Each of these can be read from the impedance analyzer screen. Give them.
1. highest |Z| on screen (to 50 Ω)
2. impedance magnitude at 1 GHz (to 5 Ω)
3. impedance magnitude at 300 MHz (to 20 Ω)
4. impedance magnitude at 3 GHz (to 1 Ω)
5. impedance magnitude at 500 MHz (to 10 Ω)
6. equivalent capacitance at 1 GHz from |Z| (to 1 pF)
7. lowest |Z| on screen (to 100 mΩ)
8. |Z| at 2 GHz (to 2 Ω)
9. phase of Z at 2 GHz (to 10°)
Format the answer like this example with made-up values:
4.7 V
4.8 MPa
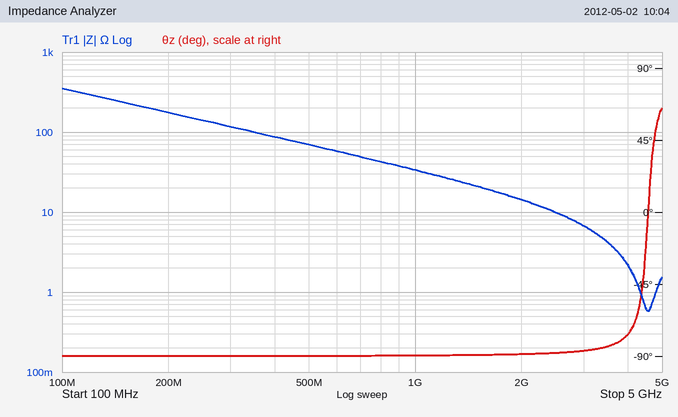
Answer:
350 Ω
35 Ω
120 Ω
7 Ω
70 Ω
5 pF
600 mΩ
14 Ω
-90°
